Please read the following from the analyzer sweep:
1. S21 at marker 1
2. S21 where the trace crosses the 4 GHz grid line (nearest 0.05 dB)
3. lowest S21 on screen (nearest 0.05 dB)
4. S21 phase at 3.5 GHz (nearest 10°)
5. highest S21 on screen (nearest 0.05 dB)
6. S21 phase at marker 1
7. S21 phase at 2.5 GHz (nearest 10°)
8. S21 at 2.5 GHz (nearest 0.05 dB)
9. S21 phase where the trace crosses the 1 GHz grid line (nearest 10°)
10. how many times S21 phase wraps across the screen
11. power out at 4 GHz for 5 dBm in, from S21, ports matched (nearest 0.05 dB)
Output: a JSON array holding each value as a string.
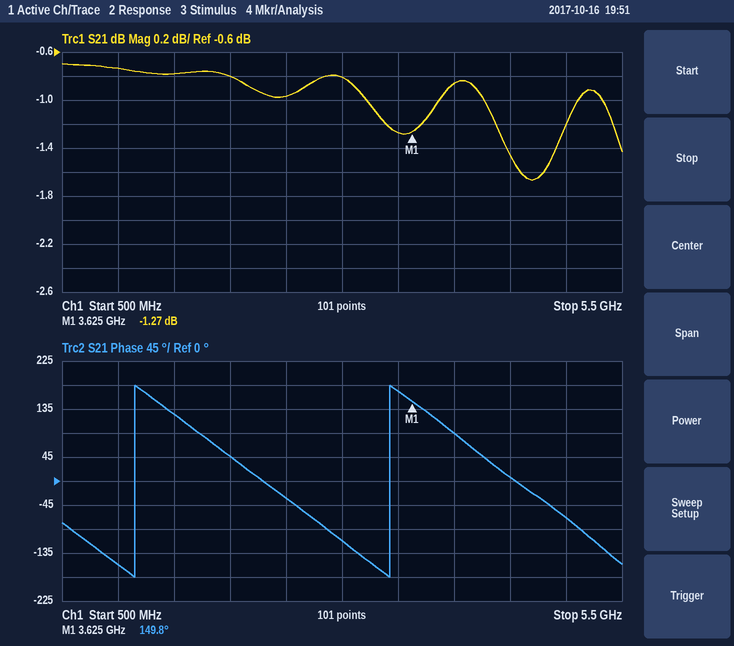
["-1.27 dB", "-0.85 dB", "-1.65 dB", "170°", "-0.70 dB", "149.8°", "-30°", "-0.95 dB", "-160°", "2", "4.15 dBm"]
